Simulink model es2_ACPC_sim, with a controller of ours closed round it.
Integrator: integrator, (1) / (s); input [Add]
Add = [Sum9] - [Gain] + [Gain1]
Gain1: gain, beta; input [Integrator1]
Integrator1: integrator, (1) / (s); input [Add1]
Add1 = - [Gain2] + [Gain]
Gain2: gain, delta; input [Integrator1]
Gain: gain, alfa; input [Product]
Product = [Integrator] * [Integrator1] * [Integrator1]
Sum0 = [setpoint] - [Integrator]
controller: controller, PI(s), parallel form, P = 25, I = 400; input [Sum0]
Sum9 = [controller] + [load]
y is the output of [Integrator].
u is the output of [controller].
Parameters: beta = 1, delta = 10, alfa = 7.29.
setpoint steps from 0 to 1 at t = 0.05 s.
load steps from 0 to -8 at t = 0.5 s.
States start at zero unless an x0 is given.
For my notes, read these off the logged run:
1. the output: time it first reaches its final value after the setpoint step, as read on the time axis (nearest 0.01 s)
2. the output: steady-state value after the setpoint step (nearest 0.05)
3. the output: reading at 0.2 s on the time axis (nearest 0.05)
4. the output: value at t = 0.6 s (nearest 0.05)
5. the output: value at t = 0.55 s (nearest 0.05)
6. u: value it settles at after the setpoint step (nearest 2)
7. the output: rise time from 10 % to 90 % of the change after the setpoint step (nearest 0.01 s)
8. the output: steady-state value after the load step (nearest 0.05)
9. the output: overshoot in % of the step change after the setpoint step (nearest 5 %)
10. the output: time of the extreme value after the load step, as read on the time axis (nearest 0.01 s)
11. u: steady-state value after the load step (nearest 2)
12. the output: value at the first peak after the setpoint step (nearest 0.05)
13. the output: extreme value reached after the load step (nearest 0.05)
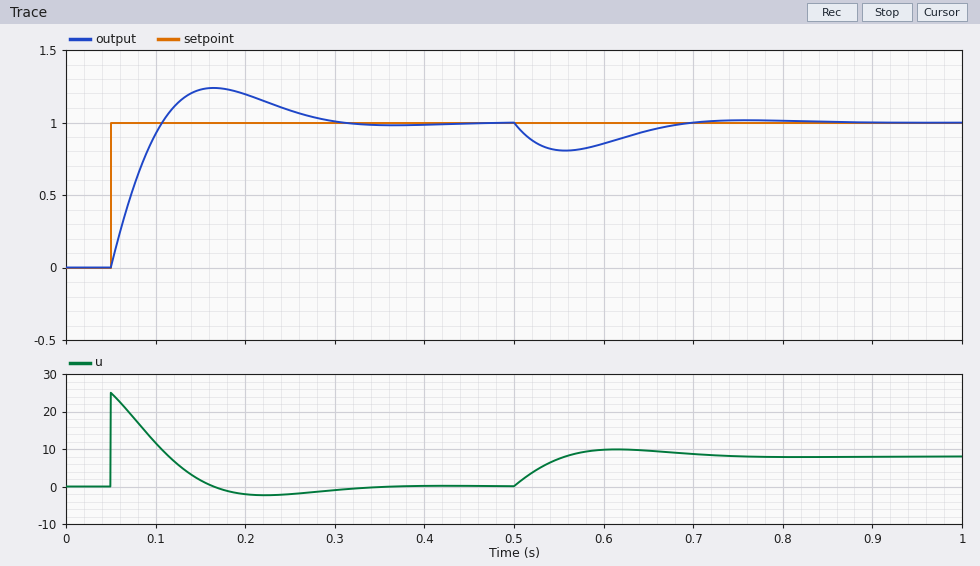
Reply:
0.11 s
1.00
1.20
0.85
0.80
0
0.04 s
1.00
25 %
0.56 s
8
1.25
0.80
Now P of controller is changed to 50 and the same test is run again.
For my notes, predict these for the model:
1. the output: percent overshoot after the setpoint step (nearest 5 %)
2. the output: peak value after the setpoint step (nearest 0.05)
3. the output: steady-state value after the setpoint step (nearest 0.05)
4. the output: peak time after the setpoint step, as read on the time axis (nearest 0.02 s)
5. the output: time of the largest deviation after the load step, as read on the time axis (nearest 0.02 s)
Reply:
10 %
1.10
1.00
0.14 s
0.54 s
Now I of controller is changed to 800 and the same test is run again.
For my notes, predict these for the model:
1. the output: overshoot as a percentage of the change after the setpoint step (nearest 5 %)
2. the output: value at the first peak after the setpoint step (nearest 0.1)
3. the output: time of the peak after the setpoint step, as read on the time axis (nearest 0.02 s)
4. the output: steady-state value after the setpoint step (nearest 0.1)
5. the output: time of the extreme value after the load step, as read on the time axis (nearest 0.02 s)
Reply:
35 %
1.3
0.14 s
1.0
0.54 s
